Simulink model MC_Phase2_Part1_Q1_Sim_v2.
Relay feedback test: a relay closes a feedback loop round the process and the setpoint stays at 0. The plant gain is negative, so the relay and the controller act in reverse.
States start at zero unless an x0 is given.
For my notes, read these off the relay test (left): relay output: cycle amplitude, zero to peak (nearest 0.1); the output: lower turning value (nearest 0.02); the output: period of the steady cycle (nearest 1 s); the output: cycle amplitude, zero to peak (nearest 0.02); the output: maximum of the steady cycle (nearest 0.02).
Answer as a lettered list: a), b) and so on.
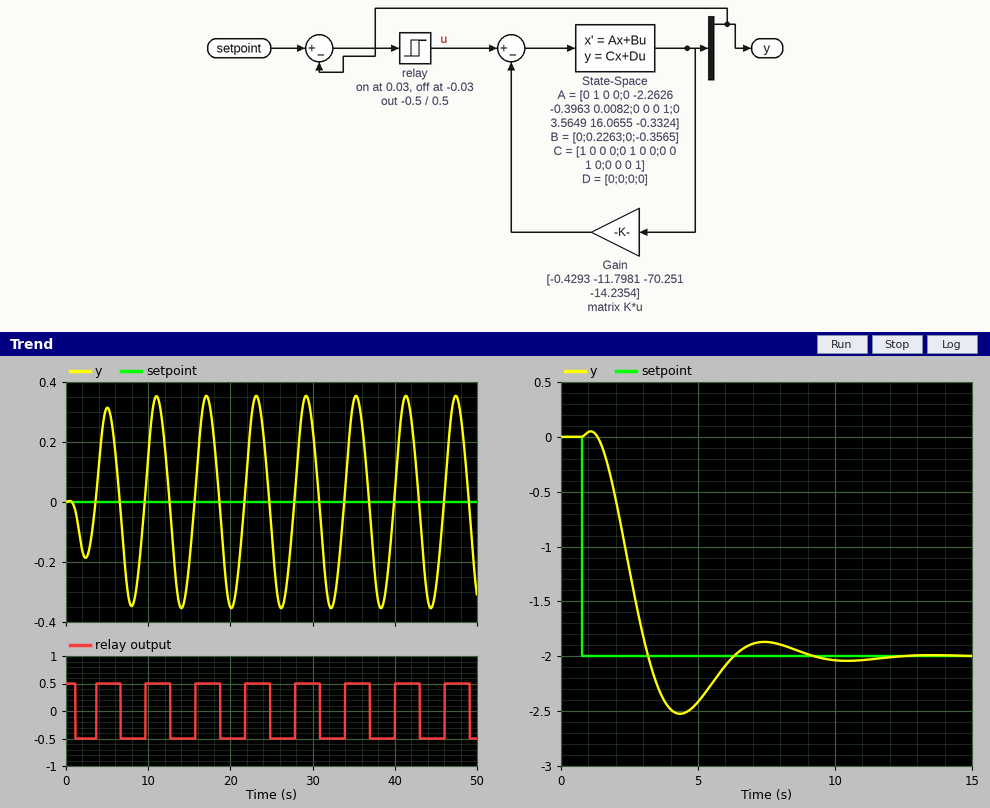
a) 0.5
b) -0.36
c) 6 s
d) 0.36
e) 0.36
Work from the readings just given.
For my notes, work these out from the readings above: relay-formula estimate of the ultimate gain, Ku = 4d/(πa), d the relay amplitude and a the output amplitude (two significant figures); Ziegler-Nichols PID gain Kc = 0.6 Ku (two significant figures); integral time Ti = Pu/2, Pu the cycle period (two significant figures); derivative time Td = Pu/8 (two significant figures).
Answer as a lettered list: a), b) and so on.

a) 1.8
b) 1.1
c) 3.0 s
d) 0.75 s
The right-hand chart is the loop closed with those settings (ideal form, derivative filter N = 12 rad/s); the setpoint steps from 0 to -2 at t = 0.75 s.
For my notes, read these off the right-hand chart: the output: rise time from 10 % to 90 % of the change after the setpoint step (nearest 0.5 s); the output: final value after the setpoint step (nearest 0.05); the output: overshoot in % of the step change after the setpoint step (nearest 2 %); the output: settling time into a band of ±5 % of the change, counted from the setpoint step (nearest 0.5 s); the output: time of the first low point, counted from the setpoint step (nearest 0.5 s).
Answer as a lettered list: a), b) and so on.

a) 1.5 s
b) -2.00
c) 26 %
d) 7.5 s
e) 3.5 s
